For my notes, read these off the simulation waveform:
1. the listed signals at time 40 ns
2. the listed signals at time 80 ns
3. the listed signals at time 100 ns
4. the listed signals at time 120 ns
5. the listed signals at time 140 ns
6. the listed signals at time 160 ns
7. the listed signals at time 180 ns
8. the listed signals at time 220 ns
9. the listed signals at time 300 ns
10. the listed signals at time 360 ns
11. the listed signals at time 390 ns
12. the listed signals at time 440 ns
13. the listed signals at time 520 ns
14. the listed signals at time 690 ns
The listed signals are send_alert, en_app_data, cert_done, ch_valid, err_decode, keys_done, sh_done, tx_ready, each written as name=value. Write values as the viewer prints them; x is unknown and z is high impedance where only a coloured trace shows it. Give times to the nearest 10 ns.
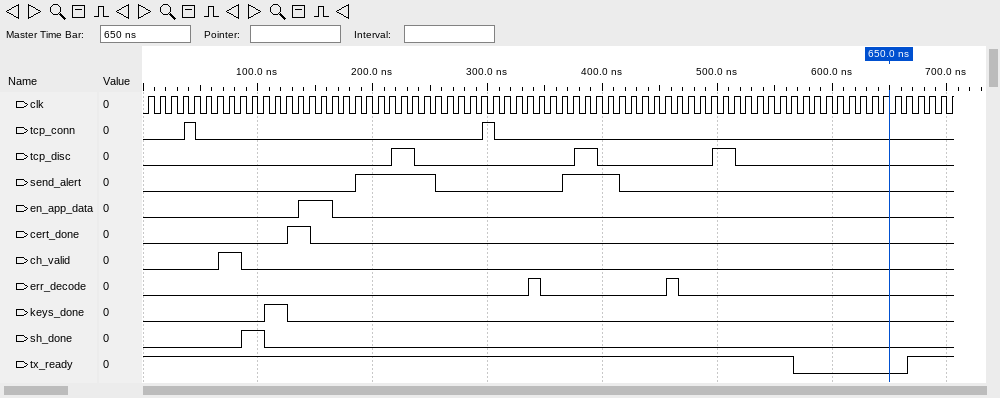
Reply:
send_alert=0, en_app_data=0, cert_done=0, ch_valid=0, err_decode=0, keys_done=0, sh_done=0, tx_ready=1
send_alert=0, en_app_data=0, cert_done=0, ch_valid=1, err_decode=0, keys_done=0, sh_done=0, tx_ready=1
send_alert=0, en_app_data=0, cert_done=0, ch_valid=0, err_decode=0, keys_done=0, sh_done=1, tx_ready=1
send_alert=0, en_app_data=0, cert_done=0, ch_valid=0, err_decode=0, keys_done=1, sh_done=0, tx_ready=1
send_alert=0, en_app_data=1, cert_done=1, ch_valid=0, err_decode=0, keys_done=0, sh_done=0, tx_ready=1
send_alert=0, en_app_data=1, cert_done=0, ch_valid=0, err_decode=0, keys_done=0, sh_done=0, tx_ready=1
send_alert=0, en_app_data=0, cert_done=0, ch_valid=0, err_decode=0, keys_done=0, sh_done=0, tx_ready=1
send_alert=1, en_app_data=0, cert_done=0, ch_valid=0, err_decode=0, keys_done=0, sh_done=0, tx_ready=1
send_alert=0, en_app_data=0, cert_done=0, ch_valid=0, err_decode=0, keys_done=0, sh_done=0, tx_ready=1
send_alert=0, en_app_data=0, cert_done=0, ch_valid=0, err_decode=0, keys_done=0, sh_done=0, tx_ready=1
send_alert=1, en_app_data=0, cert_done=0, ch_valid=0, err_decode=0, keys_done=0, sh_done=0, tx_ready=1
send_alert=0, en_app_data=0, cert_done=0, ch_valid=0, err_decode=0, keys_done=0, sh_done=0, tx_ready=1
send_alert=0, en_app_data=0, cert_done=0, ch_valid=0, err_decode=0, keys_done=0, sh_done=0, tx_ready=1
send_alert=0, en_app_data=0, cert_done=0, ch_valid=0, err_decode=0, keys_done=0, sh_done=0, tx_ready=1
